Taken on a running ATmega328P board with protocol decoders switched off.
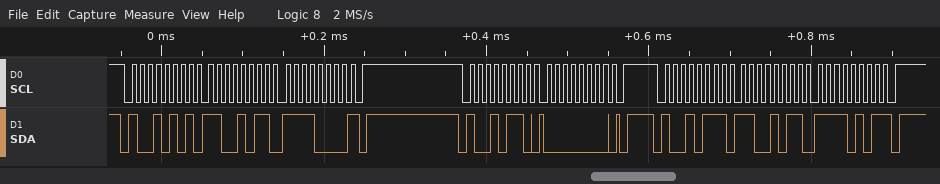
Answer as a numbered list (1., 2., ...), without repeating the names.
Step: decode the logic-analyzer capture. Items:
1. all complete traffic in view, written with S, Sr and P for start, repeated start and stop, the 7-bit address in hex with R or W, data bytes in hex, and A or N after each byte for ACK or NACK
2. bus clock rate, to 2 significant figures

1. S 4AR A CB A F0 N P S 4BW A 00 A P S 4BR A CB A F5 N P
2. 100 kHz
